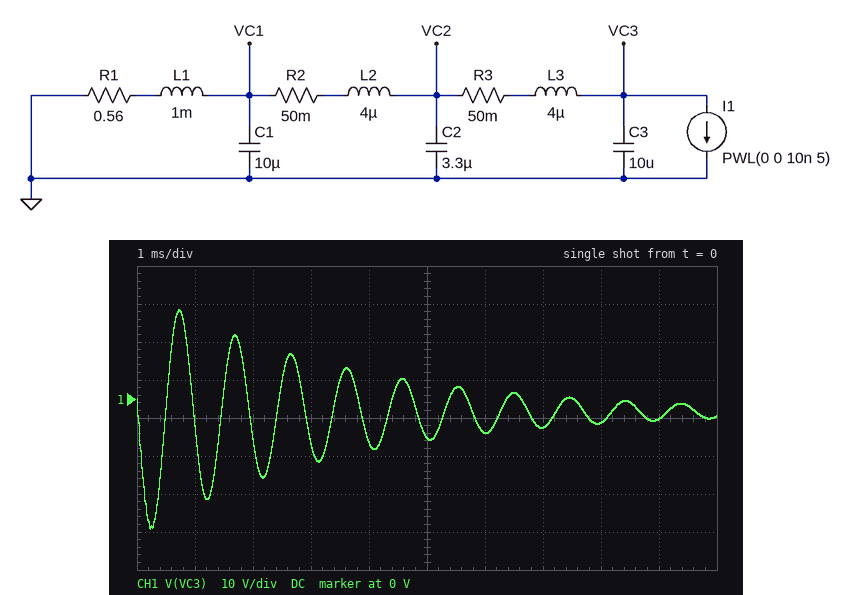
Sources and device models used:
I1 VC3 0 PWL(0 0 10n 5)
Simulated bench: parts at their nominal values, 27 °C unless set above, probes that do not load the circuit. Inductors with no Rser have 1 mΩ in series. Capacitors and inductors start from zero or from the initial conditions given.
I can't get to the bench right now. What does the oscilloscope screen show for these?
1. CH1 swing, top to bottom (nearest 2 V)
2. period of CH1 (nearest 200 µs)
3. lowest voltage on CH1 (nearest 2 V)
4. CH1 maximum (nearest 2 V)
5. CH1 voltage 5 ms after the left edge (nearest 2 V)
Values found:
58 V
1.0 ms
-34 V
24 V
-10 V
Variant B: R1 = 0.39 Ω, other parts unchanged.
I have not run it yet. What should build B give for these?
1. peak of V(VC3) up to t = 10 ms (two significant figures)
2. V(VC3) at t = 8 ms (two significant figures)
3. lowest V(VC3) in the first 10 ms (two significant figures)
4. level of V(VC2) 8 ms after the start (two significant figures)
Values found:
26 V
-8.2 V
-34 V
-7.9 V
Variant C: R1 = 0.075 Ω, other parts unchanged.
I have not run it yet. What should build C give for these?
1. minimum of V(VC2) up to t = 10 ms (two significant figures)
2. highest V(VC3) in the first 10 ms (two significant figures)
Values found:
-33 V
31 V
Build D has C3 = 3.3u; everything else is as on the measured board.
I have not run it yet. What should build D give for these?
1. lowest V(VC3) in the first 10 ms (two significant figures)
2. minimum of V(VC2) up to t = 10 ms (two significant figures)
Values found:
-41 V
-40 V
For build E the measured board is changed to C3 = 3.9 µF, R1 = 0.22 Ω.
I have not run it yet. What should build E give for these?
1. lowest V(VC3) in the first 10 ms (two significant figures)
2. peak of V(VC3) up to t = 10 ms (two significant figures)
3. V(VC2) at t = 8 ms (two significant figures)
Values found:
-40 V
34 V
13 V
